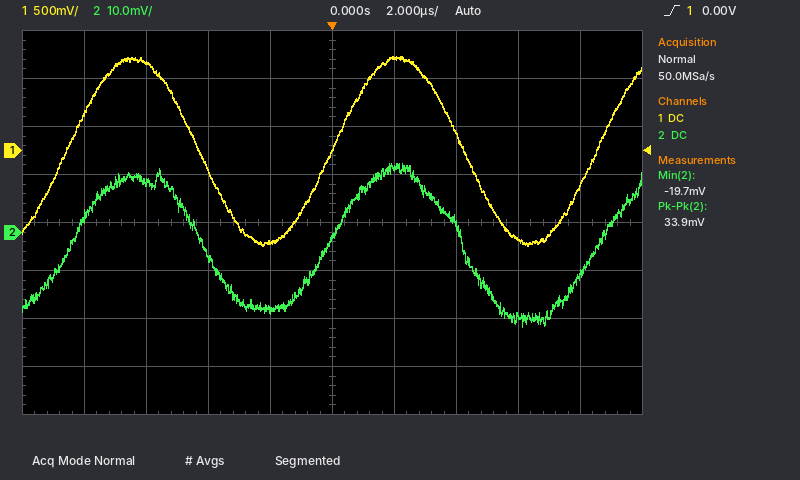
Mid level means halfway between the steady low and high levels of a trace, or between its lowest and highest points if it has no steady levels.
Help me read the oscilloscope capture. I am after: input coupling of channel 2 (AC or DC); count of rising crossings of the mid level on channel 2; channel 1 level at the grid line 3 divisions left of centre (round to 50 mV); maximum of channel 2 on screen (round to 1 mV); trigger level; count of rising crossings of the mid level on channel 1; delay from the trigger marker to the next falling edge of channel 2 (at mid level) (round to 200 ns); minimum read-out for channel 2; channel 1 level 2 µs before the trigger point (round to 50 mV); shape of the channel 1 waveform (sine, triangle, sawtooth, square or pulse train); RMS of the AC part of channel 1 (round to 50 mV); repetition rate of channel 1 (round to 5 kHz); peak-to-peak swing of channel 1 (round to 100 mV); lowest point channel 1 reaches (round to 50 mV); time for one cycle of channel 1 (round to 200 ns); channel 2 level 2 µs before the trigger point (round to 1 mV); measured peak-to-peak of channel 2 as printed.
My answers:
DC
3
900 mV
14 mV
0.00 V
3
4.2 µs
-19.7 mV
-950 mV
sine
700 mV
115 kHz
2.00 V
-1.00 V
8.6 µs
-16 mV
33.9 mV
